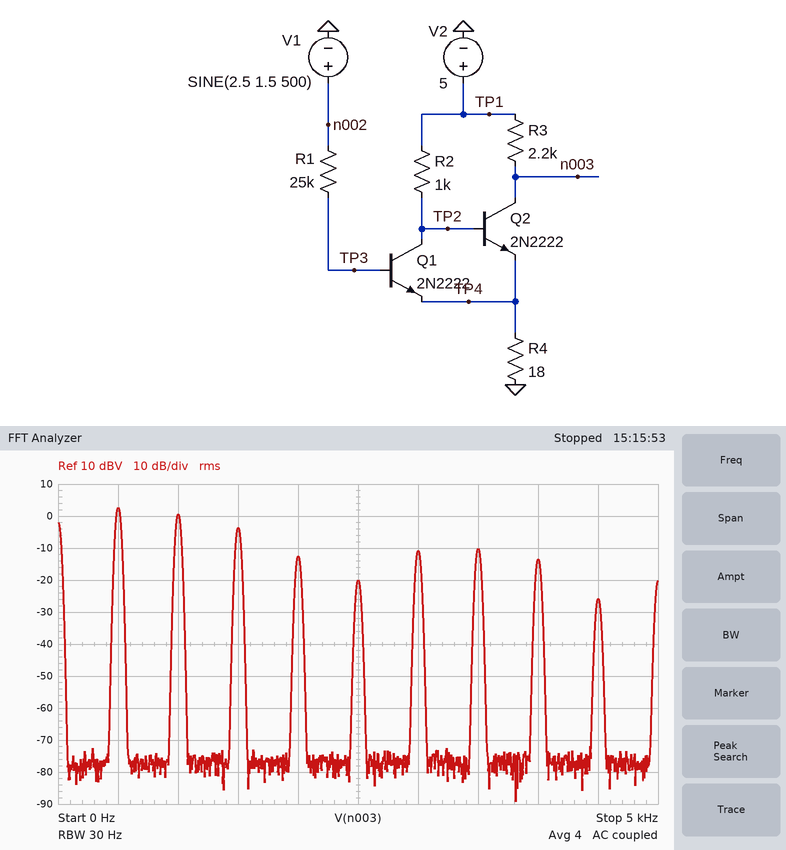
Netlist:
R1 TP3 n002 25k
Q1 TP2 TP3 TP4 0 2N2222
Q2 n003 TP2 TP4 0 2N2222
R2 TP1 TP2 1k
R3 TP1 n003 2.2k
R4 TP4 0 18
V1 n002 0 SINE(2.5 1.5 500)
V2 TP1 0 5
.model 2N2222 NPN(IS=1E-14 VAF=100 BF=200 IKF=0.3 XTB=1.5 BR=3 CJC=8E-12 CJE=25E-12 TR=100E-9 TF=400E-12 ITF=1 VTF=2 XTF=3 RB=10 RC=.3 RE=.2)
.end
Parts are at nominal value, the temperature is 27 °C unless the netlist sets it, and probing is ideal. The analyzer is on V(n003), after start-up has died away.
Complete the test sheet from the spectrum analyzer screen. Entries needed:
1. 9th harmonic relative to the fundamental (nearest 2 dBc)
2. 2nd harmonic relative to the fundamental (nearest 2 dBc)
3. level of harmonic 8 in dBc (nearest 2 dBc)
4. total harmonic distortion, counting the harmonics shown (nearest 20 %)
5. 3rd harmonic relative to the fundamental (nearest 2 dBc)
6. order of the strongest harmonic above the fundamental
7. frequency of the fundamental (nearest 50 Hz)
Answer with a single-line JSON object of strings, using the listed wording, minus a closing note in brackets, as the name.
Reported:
{"9th harmonic relative to the fundamental": "-28 dBc", "2nd harmonic relative to the fundamental": "-2 dBc", "level of harmonic 8 in dBc": "-16 dBc", "total harmonic distortion, counting the harmonics shown": "100 %", "3rd harmonic relative to the fundamental": "-6 dBc", "order of the strongest harmonic above the fundamental": "2", "frequency of the fundamental": "500 Hz"}
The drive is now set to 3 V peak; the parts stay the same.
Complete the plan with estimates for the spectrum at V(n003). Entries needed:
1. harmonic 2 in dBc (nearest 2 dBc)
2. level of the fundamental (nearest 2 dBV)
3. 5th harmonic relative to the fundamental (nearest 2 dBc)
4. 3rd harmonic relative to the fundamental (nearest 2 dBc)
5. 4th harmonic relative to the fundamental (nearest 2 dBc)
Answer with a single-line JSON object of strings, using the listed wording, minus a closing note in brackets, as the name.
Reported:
{"harmonic 2 in dBc": "-8 dBc", "level of the fundamental": "6 dBV", "5th harmonic relative to the fundamental": "-20 dBc", "3rd harmonic relative to the fundamental": "-18 dBc", "4th harmonic relative to the fundamental": "-12 dBc"}
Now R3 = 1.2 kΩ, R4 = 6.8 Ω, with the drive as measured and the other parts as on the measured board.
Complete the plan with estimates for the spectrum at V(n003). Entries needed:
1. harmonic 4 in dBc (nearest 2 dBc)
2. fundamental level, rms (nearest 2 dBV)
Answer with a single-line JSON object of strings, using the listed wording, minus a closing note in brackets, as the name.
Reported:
{"harmonic 4 in dBc": "-12 dBc", "fundamental level, rms": "2 dBV"}
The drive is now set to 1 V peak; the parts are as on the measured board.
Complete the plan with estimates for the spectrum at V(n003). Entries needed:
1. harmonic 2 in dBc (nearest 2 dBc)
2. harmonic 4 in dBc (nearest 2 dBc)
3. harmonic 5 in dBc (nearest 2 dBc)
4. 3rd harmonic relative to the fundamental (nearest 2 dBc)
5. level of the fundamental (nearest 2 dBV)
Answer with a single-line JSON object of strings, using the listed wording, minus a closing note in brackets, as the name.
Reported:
{"harmonic 2 in dBc": "-4 dBc", "harmonic 4 in dBc": "-12 dBc", "harmonic 5 in dBc": "-16 dBc", "3rd harmonic relative to the fundamental": "-8 dBc", "level of the fundamental": "-124 dBV"}
